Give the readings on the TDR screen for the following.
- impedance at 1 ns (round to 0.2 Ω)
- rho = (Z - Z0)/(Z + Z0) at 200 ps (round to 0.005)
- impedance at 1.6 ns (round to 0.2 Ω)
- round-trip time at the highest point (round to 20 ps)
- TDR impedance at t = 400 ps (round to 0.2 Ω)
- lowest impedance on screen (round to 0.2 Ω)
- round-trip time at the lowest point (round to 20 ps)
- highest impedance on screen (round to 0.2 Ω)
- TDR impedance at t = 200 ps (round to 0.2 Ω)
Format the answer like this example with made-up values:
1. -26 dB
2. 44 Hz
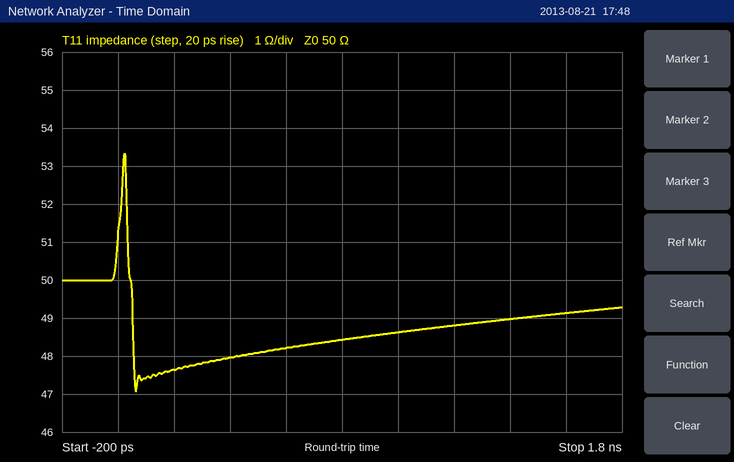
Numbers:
1. 48.6 Ω
2. -0.025
3. 49.2 Ω
4. 20 ps
5. 48.0 Ω
6. 47.0 Ω
7. 60 ps
8. 53.4 Ω
9. 47.6 Ω
